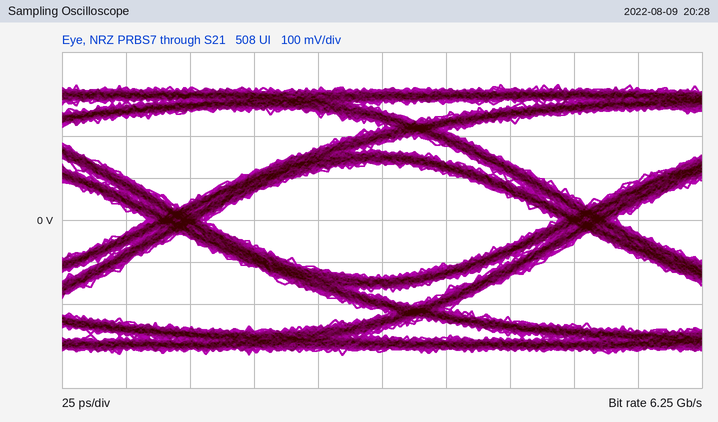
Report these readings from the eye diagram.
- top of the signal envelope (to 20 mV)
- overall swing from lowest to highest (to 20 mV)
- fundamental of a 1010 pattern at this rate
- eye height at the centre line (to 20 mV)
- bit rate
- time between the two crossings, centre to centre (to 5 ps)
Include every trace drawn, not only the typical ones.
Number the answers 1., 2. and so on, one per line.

1. 320 mV
2. 640 mV
3. 3.125 GHz
4. 280 mV
5. 6.25 Gb/s
6. 160 ps
